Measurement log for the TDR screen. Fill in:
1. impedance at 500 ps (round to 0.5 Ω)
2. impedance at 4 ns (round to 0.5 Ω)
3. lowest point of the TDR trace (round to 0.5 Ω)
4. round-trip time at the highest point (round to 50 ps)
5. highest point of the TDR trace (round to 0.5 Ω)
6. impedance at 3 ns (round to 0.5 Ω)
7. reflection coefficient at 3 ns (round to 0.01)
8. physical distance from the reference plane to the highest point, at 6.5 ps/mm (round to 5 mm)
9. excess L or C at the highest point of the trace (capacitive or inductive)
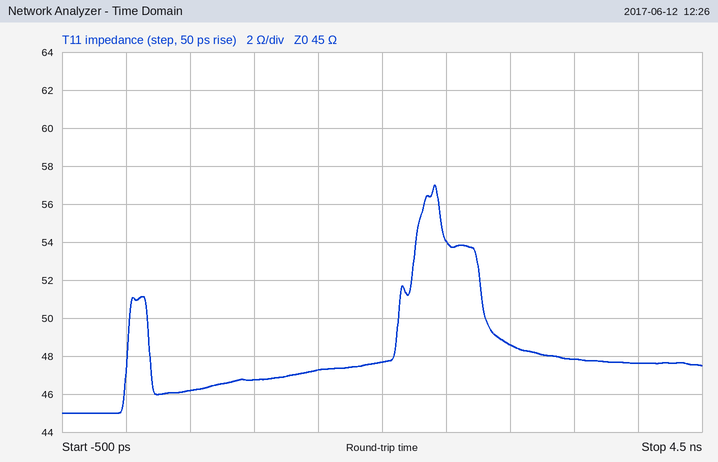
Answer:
46.0 Ω
47.5 Ω
45.0 Ω
2.40 ns
57.0 Ω
48.5 Ω
+0.04
185 mm
inductive
